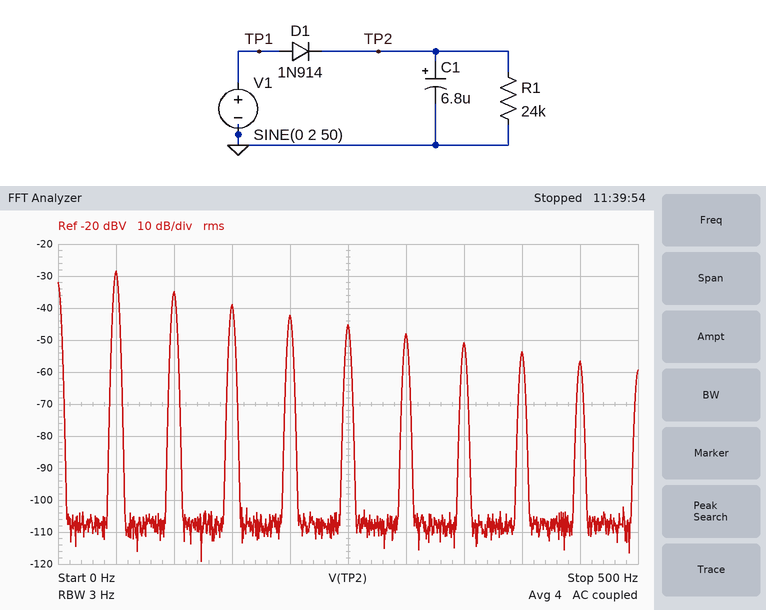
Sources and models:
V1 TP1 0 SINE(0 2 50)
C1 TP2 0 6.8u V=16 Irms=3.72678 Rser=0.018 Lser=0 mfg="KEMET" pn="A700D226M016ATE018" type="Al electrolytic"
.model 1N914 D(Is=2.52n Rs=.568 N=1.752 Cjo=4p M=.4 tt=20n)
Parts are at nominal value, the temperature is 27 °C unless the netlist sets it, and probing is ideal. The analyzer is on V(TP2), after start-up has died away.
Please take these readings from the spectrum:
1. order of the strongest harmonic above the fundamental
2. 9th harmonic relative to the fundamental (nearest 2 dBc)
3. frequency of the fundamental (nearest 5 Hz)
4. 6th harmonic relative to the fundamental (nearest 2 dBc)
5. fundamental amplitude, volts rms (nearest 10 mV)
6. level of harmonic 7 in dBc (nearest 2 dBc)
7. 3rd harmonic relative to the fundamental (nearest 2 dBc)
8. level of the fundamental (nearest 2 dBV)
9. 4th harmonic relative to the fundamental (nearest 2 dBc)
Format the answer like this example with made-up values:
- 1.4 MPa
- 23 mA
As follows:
- 2
- -28 dBc
- 50 Hz
- -20 dBc
- 40 mV
- -22 dBc
- -10 dBc
- -28 dBV
- -14 dBc
